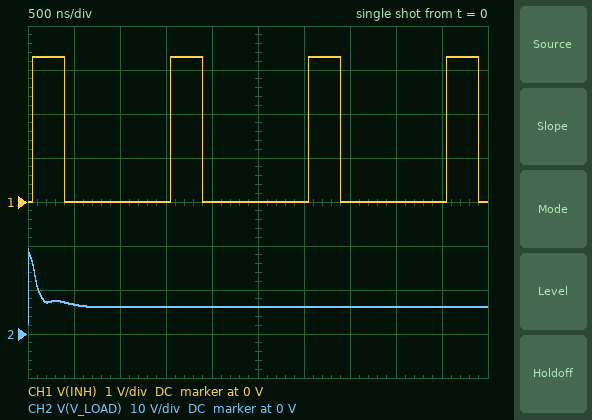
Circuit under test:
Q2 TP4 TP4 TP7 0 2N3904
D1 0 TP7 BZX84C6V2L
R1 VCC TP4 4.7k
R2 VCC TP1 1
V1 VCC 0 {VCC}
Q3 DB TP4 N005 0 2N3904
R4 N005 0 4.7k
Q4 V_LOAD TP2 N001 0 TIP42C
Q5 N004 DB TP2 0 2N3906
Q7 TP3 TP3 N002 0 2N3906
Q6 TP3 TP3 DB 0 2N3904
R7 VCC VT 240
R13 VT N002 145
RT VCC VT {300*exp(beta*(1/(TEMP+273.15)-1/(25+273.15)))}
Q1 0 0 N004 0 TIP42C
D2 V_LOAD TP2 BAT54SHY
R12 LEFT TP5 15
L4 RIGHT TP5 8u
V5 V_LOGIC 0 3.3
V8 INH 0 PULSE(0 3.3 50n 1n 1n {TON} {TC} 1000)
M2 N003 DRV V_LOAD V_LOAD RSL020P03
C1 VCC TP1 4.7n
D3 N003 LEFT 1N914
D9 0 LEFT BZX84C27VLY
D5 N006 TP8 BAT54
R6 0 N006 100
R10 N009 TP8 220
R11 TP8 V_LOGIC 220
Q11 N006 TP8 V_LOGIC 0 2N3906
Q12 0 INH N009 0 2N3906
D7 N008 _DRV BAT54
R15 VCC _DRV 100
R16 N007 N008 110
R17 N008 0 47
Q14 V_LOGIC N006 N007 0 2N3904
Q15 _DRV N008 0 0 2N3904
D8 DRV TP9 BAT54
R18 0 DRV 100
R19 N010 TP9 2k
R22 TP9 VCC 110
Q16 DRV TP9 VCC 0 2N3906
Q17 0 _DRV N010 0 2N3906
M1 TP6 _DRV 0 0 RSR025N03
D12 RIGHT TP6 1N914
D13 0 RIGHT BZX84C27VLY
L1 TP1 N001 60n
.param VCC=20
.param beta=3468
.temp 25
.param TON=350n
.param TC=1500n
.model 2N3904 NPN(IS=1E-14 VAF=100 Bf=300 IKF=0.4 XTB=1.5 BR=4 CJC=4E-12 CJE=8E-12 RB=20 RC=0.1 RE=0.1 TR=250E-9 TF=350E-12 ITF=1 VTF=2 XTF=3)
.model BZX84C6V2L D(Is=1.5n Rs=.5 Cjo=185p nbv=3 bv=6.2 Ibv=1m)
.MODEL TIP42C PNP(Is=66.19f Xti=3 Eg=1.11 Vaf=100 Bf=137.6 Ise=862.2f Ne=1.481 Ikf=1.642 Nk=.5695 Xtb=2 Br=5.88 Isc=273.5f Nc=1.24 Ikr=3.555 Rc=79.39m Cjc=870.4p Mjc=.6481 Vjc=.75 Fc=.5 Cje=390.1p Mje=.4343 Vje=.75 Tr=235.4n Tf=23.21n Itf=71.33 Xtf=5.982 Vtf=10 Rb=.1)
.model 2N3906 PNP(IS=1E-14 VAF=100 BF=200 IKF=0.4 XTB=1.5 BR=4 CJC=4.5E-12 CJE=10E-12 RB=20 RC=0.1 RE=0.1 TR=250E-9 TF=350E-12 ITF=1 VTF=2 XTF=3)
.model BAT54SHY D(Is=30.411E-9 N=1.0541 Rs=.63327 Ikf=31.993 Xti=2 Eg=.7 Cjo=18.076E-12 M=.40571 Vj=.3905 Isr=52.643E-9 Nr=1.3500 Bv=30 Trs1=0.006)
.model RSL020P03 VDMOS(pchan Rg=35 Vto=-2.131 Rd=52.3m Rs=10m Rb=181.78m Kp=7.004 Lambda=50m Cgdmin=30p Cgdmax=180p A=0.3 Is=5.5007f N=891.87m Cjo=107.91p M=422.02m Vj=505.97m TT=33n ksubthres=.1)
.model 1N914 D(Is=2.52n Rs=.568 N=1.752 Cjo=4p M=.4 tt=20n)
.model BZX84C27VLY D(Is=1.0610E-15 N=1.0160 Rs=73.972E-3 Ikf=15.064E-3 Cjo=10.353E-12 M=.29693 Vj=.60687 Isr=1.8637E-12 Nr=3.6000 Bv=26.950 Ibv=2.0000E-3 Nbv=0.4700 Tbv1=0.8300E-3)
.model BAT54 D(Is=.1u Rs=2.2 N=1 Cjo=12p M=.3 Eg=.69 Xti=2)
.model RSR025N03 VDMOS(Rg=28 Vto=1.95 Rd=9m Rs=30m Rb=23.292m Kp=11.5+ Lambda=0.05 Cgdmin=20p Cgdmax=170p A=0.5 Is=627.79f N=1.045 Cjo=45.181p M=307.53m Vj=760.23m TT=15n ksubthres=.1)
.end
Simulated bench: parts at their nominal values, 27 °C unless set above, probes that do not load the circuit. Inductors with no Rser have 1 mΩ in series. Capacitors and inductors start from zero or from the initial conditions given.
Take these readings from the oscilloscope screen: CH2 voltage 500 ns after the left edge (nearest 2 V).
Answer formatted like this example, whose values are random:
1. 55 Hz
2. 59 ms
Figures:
1. 6 V
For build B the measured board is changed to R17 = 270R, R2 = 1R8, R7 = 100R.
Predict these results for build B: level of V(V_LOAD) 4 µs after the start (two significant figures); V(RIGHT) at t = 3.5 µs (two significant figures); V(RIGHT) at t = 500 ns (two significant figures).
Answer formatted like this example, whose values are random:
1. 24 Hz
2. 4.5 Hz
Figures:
1. 20 V
2. 970 mV
3. 930 mV
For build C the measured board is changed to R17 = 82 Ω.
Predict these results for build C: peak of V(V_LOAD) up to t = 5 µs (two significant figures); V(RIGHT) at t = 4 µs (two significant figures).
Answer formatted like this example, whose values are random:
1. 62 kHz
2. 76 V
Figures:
1. 20 V
2. 27 V
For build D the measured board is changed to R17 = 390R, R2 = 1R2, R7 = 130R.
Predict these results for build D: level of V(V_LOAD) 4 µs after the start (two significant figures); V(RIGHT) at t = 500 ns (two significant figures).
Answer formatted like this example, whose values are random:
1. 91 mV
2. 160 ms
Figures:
1. 20 V
2. 950 mV
